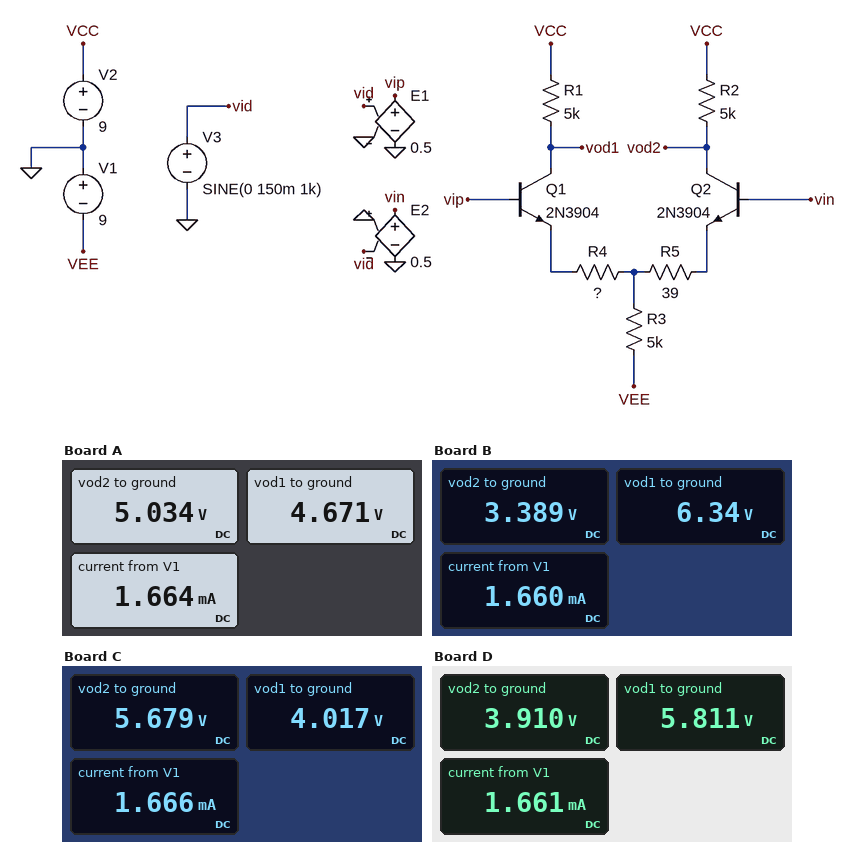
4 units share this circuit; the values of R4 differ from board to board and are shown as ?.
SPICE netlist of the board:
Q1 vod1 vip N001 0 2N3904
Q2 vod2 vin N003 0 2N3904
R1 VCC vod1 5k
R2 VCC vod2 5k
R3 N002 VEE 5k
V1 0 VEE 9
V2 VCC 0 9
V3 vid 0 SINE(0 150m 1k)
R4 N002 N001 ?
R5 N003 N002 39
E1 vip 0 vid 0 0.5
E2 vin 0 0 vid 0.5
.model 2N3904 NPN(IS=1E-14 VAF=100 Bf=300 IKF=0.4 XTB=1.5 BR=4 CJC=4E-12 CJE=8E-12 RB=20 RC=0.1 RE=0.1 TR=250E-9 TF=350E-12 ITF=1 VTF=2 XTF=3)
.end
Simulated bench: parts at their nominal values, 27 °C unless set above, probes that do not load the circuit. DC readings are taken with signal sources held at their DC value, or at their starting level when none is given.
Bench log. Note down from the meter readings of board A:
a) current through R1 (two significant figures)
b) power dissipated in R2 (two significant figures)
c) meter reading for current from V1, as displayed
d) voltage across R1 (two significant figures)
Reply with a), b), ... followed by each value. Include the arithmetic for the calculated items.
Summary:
a) (9 V - 4.671 V) / 5 kΩ = 870 µA
b) (9 V - 5.034 V)^2 / 5 kΩ = 3.1 mW
c) 1.664 mA
d) 9 V - 4.671 V = 4.3 V
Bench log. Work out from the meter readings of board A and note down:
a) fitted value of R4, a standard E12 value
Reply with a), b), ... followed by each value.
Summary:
a) 33 Ω
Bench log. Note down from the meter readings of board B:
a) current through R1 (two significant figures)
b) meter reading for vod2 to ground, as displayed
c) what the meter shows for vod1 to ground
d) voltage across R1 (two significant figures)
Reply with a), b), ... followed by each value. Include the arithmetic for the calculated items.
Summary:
a) (9 V - 6.34 V) / 5 kΩ = 530 µA
b) 3.389 V
c) 6.34 V
d) 9 V - 6.34 V = 2.7 V
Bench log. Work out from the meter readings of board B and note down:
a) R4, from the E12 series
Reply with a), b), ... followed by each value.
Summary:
a) 120 Ω
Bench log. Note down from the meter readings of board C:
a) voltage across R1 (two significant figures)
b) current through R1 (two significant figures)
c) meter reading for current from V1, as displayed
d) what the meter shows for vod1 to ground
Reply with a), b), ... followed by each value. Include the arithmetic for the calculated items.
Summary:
a) 9 V - 4.017 V = 5.0 V
b) (9 V - 4.017 V) / 5 kΩ = 1.0 mA
c) 1.666 mA
d) 4.017 V
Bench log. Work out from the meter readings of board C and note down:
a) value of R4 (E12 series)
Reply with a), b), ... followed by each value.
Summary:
a) 15 Ω
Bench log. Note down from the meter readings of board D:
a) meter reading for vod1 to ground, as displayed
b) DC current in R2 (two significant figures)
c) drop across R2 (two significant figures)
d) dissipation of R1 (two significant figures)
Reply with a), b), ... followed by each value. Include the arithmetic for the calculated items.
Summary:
a) 5.811 V
b) (9 V - 3.91 V) / 5 kΩ = 1.0 mA
c) 9 V - 3.91 V = 5.1 V
d) (9 V - 5.811 V)^2 / 5 kΩ = 2.0 mW
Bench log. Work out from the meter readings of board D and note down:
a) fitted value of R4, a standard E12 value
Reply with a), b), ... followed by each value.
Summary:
a) 82 Ω
